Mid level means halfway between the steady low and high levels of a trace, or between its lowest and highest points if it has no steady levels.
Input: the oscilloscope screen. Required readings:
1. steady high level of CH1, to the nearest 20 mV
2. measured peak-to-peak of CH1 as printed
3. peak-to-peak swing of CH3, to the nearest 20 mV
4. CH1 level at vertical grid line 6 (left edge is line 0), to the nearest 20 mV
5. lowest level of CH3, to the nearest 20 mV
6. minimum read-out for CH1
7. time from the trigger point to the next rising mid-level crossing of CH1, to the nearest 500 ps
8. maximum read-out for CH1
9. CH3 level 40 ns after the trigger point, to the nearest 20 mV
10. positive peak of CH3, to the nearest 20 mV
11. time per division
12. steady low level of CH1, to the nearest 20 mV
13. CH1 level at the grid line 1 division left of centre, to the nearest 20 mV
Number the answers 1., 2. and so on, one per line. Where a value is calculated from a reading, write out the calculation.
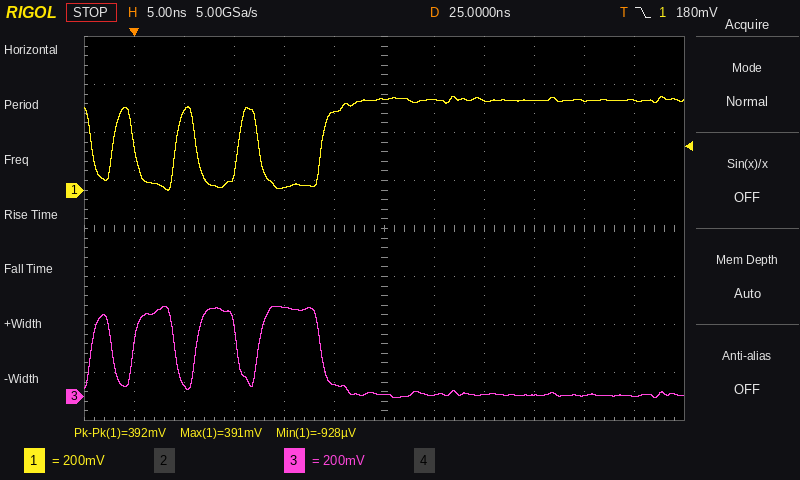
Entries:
1. 380 mV
2. 392 mV
3. 380 mV − (0 mV) = 380 mV
4. 380 mV
5. 0 mV
6. -928 µV
7. 4.0 ns
8. 391 mV
9. 0 mV
10. 380 mV
11. 5 ns
12. 20 mV
13. 320 mV
